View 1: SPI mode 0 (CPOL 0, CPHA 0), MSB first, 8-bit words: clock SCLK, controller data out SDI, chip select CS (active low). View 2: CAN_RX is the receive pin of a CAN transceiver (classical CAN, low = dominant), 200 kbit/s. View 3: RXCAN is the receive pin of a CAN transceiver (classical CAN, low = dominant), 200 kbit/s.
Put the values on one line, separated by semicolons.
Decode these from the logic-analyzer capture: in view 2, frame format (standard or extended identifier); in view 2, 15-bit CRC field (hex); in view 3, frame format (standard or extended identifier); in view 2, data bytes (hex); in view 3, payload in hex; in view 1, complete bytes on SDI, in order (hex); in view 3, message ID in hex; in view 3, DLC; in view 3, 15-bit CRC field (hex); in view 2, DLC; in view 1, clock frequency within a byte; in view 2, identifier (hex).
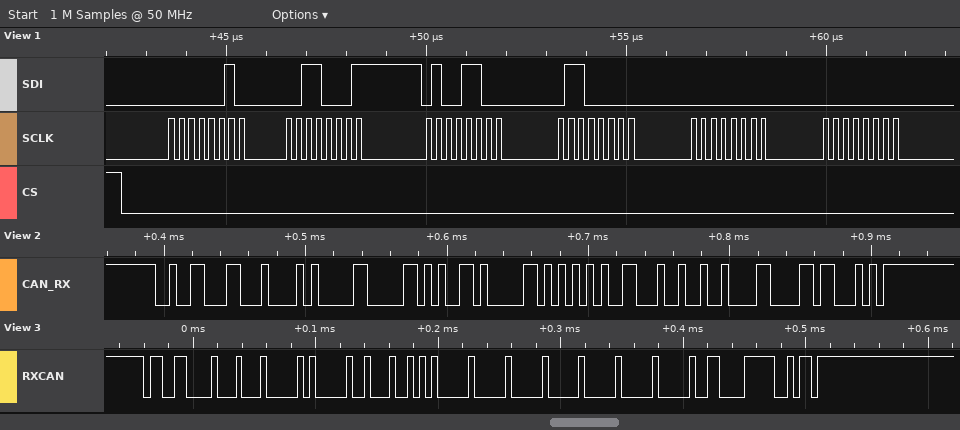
standard; 0x4362; standard; 50 41 53 41 55 4C 49 21; 81 01 12 A0 00 00 00 00; 0x02 0x31 0x4C 0x60 0x00 0x00; 0x661; 8; 0x61F5; 8; 4 MHz; 0x263
